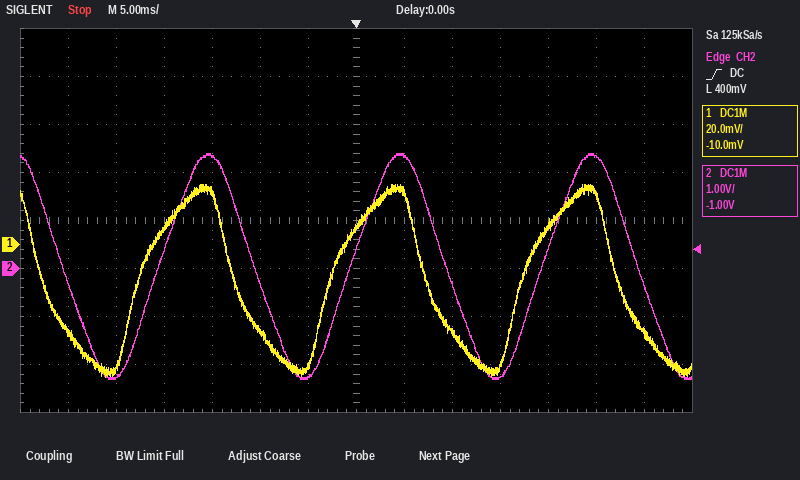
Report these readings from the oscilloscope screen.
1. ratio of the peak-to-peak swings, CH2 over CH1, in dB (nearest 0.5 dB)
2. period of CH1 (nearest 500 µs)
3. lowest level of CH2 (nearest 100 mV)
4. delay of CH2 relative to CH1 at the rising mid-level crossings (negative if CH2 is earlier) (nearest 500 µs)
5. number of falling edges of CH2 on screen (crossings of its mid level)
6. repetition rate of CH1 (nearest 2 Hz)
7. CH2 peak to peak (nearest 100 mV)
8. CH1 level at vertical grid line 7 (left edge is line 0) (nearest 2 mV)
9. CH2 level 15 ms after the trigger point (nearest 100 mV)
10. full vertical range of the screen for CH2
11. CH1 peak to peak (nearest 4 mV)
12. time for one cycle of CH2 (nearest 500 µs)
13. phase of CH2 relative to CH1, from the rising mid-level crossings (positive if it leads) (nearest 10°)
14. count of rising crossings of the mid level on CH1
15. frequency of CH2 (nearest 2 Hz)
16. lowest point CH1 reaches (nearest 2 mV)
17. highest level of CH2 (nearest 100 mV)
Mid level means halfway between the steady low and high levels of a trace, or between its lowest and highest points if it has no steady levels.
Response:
35.5 dB
20.0 ms
-2.3 V
+2.0 ms
4
50 Hz
4.7 V
6 mV
-2.3 V
8 V
80 mV
20.0 ms
-40°
3
50 Hz
-56 mV
2.4 V
